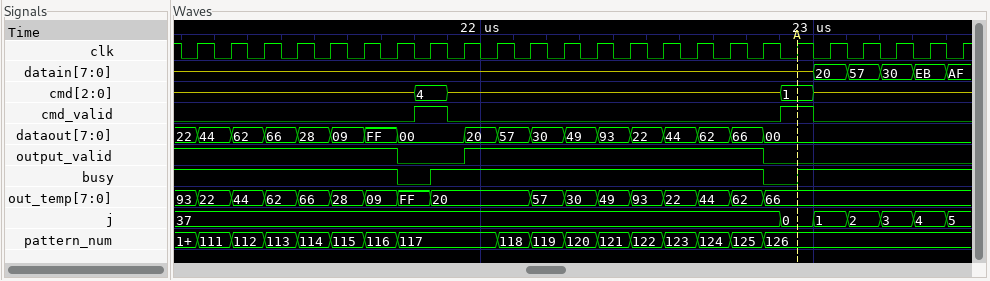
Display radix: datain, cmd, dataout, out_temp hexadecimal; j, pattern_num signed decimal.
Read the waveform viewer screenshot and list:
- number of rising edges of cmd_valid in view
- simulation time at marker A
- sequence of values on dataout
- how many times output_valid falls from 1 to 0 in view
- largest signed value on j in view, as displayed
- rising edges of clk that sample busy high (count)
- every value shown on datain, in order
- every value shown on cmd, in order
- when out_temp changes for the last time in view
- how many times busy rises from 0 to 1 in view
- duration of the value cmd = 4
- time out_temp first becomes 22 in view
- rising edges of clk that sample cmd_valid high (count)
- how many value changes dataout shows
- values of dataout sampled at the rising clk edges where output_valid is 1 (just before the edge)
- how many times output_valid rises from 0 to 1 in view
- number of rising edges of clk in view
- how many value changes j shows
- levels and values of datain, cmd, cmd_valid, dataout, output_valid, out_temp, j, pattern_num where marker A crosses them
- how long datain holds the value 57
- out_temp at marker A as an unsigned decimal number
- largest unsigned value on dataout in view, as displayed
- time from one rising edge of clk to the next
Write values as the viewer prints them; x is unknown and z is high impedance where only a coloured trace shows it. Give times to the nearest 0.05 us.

2
22.95 us
22, 44, 62, 66, 28, 09, FF, 00, 20, 57, 30, 49, 93, 22, 44, 62, 66, 00
2
37
22
z, 20, 57, 30, EB, AF
z, 4, z, 1, z
22.85 us
2
0.1 us
21.15 us
2
17
22, 44, 62, 66, 28, 09, FF, 20, 57, 30, 49, 93, 22, 44, 62, 66
1
24
6
datain=z, cmd=1, cmd_valid=1, dataout=00, output_valid=0, out_temp=66, j=0, pattern_num=126
0.1 us
102
FF
0.1 us
